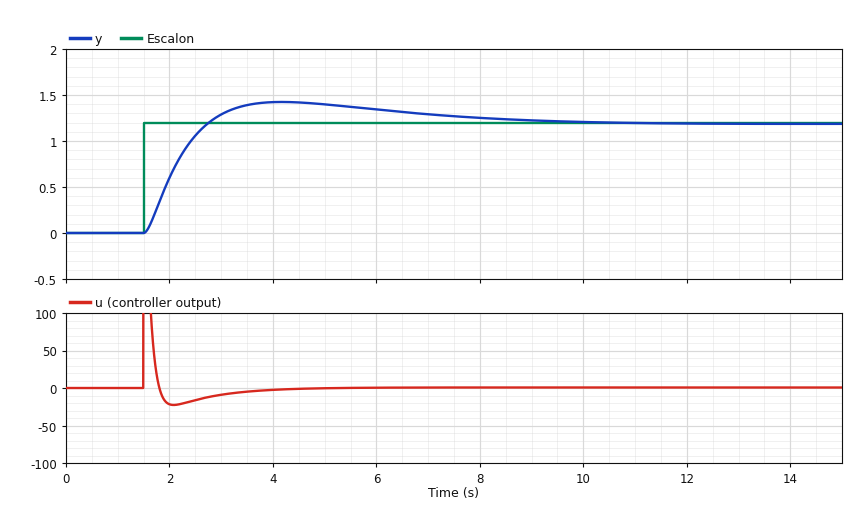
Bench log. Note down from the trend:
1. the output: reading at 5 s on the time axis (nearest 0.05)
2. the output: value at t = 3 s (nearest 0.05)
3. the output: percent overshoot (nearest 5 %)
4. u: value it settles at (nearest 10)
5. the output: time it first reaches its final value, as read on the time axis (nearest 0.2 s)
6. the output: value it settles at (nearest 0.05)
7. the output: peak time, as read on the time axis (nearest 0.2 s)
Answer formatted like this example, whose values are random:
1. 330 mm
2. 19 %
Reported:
1. 1.40
2. 1.30
3. 20 %
4. 0
5. 2.8 s
6. 1.20
7. 4.2 s
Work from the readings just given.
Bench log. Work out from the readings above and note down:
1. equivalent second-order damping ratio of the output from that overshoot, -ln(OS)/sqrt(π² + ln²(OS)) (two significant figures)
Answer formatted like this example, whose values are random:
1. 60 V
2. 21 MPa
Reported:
1. 0.46
